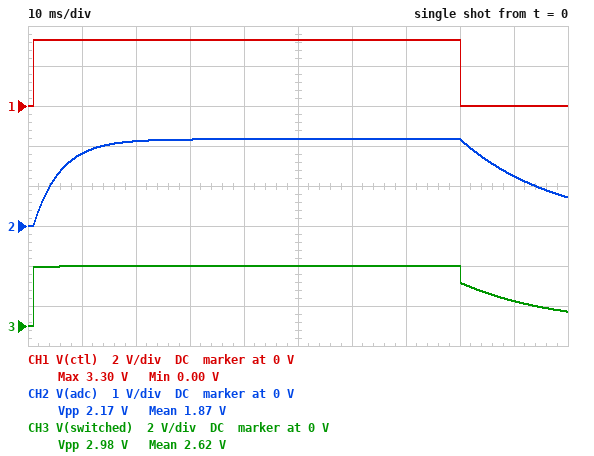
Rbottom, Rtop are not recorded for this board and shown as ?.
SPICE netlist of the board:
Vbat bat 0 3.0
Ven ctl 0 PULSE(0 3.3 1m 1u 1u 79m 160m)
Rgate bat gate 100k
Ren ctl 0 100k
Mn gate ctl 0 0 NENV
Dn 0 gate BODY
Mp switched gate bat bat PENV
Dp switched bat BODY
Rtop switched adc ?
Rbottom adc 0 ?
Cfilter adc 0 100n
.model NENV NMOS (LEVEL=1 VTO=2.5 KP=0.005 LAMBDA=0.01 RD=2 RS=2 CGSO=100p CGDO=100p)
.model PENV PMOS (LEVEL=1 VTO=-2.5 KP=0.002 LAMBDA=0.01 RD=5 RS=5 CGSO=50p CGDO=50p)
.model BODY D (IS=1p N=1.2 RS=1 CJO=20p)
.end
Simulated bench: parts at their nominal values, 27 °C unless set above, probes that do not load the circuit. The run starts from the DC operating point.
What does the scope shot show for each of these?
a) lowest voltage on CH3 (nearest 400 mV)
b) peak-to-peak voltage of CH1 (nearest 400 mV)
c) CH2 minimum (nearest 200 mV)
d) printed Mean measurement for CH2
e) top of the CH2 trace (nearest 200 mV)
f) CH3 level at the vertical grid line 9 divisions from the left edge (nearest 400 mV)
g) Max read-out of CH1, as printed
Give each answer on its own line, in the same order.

0 V
3.2 V
0 V
1.87 V
2.2 V
1.2 V
3.30 V
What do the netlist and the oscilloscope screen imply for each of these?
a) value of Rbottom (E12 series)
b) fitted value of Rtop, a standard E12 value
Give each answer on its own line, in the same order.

180 kΩ
68 kΩ
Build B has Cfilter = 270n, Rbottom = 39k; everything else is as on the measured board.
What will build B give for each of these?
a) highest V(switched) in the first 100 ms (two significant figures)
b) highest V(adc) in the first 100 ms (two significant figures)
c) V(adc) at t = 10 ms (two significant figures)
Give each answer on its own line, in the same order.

3.0 V
1.1 V
800 mV
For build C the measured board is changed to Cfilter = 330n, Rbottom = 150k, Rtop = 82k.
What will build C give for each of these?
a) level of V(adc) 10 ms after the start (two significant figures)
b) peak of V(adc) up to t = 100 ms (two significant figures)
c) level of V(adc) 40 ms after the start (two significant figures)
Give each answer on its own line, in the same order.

770 mV
1.9 V
1.7 V
